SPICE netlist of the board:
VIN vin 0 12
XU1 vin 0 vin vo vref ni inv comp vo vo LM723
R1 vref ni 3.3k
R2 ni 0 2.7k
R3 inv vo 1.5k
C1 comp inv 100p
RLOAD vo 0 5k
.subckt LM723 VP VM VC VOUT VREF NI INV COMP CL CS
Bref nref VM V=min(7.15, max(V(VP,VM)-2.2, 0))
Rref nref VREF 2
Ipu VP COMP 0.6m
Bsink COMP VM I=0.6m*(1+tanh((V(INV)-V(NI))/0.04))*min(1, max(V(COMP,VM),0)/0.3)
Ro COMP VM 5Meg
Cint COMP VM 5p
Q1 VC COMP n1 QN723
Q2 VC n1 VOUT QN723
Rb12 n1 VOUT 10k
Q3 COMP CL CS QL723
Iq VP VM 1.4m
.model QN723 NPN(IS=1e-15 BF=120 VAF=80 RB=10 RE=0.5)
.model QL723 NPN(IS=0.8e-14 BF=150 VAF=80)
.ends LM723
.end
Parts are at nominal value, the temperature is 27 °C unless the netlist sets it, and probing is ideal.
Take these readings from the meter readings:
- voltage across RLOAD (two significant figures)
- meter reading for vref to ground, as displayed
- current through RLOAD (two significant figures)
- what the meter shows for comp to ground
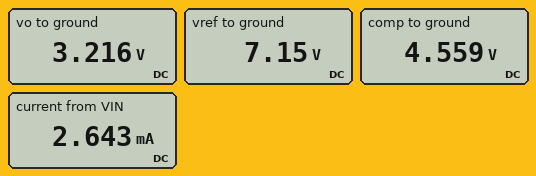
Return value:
3.2 V
7.15 V
640 µA
4.559 V
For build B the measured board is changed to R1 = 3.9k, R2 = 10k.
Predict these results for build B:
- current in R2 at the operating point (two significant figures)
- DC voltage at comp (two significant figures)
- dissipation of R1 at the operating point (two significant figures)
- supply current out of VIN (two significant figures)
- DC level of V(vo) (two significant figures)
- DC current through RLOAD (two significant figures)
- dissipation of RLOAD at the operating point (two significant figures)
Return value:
510 µA
6.5 V
1.0 mW
3.0 mA
5.1 V
1.0 mA
5.3 mW
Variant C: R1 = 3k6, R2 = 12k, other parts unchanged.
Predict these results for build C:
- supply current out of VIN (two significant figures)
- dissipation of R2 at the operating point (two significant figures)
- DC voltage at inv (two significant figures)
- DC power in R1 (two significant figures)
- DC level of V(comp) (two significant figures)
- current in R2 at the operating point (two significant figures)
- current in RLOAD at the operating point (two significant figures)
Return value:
3.1 mA
2.5 mW
5.5 V
760 µW
6.9 V
460 µA
1.1 mA
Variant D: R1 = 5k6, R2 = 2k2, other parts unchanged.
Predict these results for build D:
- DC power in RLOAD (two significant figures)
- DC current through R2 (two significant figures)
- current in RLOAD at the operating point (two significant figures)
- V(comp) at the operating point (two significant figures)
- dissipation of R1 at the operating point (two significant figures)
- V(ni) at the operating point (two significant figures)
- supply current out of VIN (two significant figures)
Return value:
810 µW
920 µA
400 µA
3.3 V
4.7 mW
2.0 V
2.4 mA
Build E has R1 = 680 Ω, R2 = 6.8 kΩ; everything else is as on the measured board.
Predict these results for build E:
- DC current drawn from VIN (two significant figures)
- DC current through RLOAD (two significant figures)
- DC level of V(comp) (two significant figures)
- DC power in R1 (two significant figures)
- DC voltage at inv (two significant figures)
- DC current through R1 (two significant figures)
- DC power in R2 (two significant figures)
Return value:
3.3 mA
1.3 mA
7.9 V
620 µW
6.5 V
960 µA
6.2 mW
